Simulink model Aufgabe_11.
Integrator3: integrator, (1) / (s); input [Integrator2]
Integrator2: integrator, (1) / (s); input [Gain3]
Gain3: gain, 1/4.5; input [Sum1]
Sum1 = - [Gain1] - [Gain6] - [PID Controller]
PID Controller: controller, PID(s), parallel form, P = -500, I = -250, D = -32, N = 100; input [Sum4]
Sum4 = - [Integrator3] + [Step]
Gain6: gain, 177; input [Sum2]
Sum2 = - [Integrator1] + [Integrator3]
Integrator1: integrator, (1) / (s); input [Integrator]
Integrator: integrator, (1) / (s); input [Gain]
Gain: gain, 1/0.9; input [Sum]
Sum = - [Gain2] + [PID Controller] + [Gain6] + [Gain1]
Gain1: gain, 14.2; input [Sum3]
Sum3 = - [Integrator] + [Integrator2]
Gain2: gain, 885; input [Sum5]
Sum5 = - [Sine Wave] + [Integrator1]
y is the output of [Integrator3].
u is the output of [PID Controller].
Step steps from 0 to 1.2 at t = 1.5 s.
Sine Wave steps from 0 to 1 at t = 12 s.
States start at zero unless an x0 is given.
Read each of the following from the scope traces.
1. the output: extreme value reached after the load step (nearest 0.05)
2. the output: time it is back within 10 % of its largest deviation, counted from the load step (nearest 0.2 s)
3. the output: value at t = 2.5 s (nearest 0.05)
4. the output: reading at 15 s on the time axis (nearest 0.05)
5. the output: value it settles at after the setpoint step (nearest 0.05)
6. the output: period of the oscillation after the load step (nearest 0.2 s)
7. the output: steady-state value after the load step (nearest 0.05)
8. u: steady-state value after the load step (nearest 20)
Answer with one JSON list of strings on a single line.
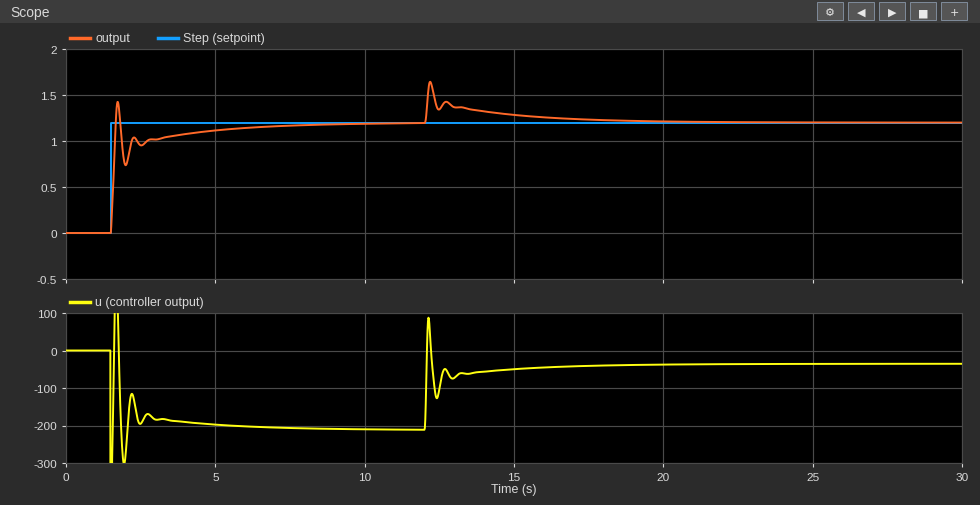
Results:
["1.65", "4.6 s", "0.95", "1.30", "1.20", "0.6 s", "1.20", "-40"]
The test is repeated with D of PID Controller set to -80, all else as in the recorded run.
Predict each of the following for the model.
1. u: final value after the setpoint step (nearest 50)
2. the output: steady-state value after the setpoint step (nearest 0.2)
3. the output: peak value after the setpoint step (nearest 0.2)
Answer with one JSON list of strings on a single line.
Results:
["-200", "1.2", "1.4"]
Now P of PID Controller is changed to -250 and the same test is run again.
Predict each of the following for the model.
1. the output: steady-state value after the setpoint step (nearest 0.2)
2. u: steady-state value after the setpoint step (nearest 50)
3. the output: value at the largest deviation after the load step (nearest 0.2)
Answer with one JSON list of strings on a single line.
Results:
["1.2", "-200", "1.8"]
